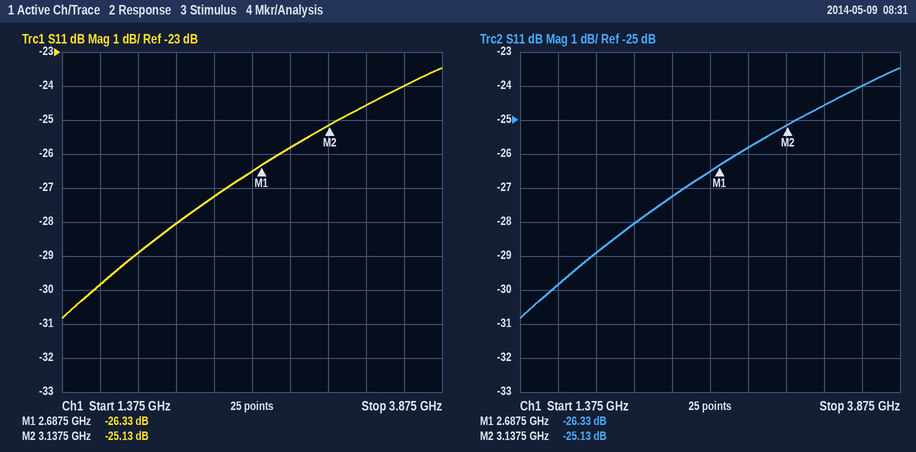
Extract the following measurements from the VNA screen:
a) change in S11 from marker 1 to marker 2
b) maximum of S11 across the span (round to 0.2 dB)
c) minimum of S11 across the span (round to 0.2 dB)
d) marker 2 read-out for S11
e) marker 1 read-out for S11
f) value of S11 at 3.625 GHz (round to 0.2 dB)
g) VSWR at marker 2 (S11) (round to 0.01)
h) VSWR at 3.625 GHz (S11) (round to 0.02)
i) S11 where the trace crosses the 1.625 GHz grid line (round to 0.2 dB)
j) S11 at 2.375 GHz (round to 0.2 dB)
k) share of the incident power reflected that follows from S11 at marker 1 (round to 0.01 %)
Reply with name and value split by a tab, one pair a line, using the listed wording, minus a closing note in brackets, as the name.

change in S11 from marker 1 to marker 2	1.20 dB
maximum of S11 across the span	-23.4 dB
minimum of S11 across the span	-30.8 dB
marker 2 read-out for S11	-25.13 dB
marker 1 read-out for S11	-26.33 dB
value of S11 at 3.625 GHz	-24.0 dB
VSWR at marker 2 (S11)	1.12
VSWR at 3.625 GHz (S11)	1.14
S11 where the trace crosses the 1.625 GHz grid line	-29.8 dB
S11 at 2.375 GHz	-27.2 dB
share of the incident power reflected that follows from S11 at marker 1	0.23 %
